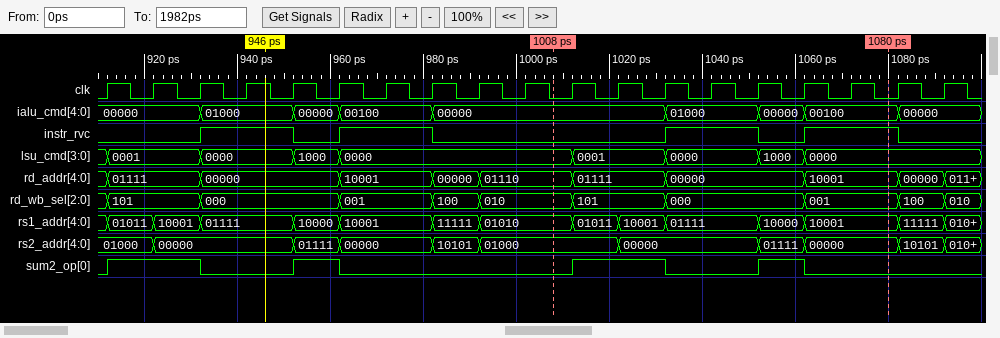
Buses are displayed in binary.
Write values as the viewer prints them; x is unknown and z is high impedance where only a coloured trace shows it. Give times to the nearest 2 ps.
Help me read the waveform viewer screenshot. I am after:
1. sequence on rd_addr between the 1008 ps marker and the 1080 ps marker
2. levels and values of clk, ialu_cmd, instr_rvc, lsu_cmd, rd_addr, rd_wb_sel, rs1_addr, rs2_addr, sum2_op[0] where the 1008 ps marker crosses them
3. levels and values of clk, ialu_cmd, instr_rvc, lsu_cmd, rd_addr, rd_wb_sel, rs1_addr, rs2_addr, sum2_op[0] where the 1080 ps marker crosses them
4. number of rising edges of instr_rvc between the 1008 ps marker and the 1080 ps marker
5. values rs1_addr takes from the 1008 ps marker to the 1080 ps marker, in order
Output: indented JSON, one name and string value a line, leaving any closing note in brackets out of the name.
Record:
{
  "sequence on rd_addr between the 1008 ps marker and the 1080 ps marker": "01110, 01111, 00000, 10001",
  "levels and values of clk, ialu_cmd, instr_rvc, lsu_cmd, rd_addr, rd_wb_sel, rs1_addr, rs2_addr, sum2_op[0] where the 1008 ps marker crosses them": "clk=0, ialu_cmd=00000, instr_rvc=0, lsu_cmd=0000, rd_addr=01110, rd_wb_sel=010, rs1_addr=01010, rs2_addr=01000, sum2_op[0]=0",
  "levels and values of clk, ialu_cmd, instr_rvc, lsu_cmd, rd_addr, rd_wb_sel, rs1_addr, rs2_addr, sum2_op[0] where the 1080 ps marker crosses them": "clk=0, ialu_cmd=00100, instr_rvc=1, lsu_cmd=0000, rd_addr=10001, rd_wb_sel=001, rs1_addr=10001, rs2_addr=00000, sum2_op[0]=0",
  "number of rising edges of instr_rvc between the 1008 ps marker and the 1080 ps marker": "2",
  "values rs1_addr takes from the 1008 ps marker to the 1080 ps marker, in order": "01010, 01011, 10001, 01111, 10000, 10001"
}
